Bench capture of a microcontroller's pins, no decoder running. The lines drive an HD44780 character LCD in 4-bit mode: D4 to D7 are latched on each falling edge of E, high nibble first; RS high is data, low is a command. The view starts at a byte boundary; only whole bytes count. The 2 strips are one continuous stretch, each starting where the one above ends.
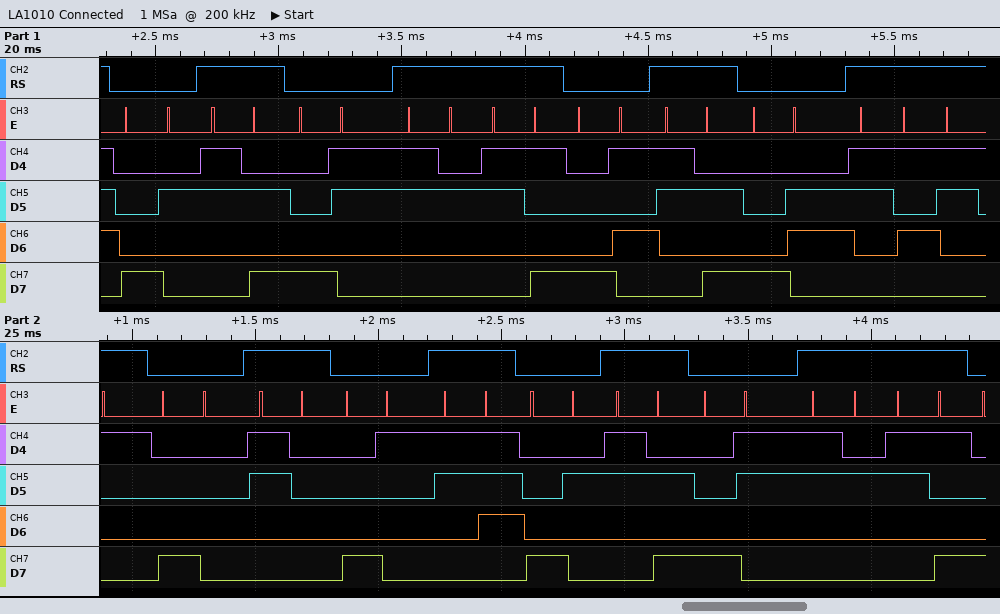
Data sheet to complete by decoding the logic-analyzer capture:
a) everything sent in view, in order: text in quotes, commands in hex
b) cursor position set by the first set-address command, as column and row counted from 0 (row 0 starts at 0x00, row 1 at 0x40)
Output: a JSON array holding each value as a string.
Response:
["0x82 \":\" 0x83 \"29\" 0x85 \":\" 0x86 \"51\" 0x80 \"0\" 0x81 \"7\" 0x82 \":\" 0x83 \"29\"", "column 2, row 0"]
